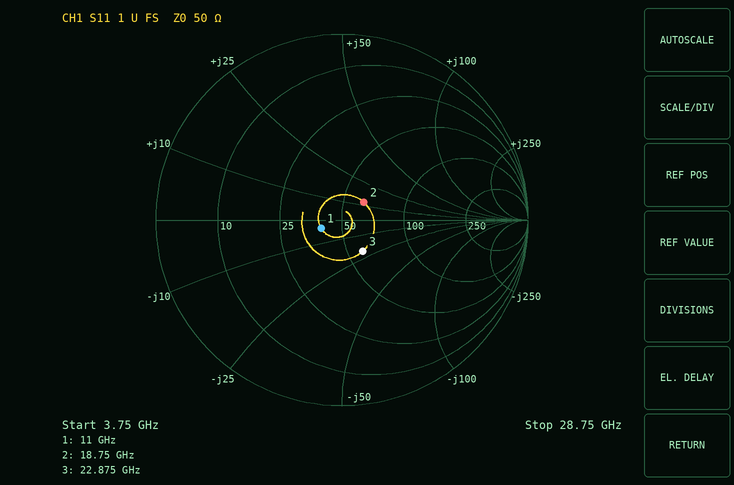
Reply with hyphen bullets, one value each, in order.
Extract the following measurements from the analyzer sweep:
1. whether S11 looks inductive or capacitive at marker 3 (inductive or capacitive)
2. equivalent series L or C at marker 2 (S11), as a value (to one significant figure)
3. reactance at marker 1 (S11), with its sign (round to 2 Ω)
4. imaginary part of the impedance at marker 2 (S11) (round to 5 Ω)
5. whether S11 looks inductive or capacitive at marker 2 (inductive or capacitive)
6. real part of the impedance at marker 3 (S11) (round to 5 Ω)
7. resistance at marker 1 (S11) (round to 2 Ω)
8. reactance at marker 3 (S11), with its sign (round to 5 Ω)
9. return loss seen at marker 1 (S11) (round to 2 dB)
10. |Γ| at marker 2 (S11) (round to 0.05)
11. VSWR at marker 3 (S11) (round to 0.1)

- capacitive
- 100 pH
- -4 Ω
- +10 Ω
- inductive
- 60 Ω
- 40 Ω
- -20 Ω
- 18 dB
- 0.15
- 1.5
